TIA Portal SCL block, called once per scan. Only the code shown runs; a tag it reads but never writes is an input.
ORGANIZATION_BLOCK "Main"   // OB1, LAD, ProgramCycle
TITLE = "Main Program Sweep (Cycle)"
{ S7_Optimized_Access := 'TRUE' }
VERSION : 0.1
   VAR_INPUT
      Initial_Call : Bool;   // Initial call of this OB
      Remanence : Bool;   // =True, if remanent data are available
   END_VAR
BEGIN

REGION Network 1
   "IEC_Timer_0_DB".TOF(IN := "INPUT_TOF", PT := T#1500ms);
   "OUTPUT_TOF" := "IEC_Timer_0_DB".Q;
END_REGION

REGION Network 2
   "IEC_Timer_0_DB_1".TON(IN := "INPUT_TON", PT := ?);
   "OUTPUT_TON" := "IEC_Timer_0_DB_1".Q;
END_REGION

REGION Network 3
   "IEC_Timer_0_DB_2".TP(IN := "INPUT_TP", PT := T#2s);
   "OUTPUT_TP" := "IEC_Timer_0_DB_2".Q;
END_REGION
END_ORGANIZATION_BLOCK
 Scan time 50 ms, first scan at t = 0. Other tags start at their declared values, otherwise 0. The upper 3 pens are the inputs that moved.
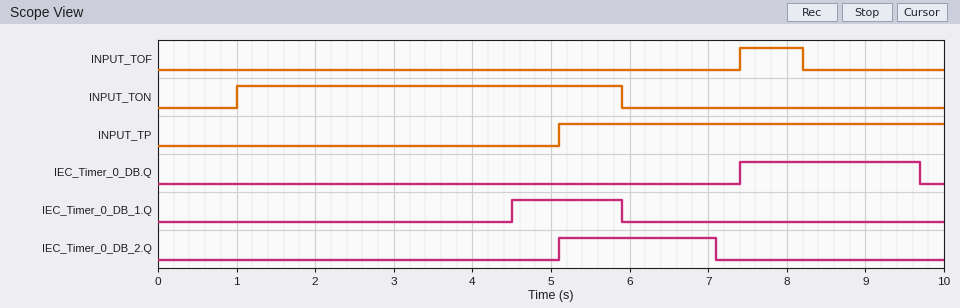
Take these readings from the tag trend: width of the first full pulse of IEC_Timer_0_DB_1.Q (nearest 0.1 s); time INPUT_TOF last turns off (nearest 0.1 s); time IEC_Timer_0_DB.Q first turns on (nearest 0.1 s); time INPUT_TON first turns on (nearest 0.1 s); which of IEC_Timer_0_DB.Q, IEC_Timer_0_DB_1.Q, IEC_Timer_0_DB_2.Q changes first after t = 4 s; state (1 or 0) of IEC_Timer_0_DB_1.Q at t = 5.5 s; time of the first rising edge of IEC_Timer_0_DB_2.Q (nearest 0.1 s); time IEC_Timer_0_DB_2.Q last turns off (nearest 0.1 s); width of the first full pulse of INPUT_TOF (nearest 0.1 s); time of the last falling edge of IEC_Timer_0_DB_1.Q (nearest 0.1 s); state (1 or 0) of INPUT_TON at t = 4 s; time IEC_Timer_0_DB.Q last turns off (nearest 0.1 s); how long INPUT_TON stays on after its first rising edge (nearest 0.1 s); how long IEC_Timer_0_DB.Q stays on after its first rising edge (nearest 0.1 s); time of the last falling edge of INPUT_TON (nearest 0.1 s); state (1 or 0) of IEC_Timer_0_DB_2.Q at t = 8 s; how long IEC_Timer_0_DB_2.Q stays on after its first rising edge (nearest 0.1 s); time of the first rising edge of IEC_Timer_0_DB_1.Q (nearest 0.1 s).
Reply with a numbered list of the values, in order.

1. 1.4 s
2. 8.2 s
3. 7.4 s
4. 1.0 s
5. IEC_Timer_0_DB_1.Q
6. 1
7. 5.1 s
8. 7.1 s
9. 0.8 s
10. 5.9 s
11. 1
12. 9.7 s
13. 4.9 s
14. 2.3 s
15. 5.9 s
16. 0
17. 2.0 s
18. 4.5 s
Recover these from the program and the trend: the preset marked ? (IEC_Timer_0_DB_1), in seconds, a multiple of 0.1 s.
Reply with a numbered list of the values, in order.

1. 3.5 s
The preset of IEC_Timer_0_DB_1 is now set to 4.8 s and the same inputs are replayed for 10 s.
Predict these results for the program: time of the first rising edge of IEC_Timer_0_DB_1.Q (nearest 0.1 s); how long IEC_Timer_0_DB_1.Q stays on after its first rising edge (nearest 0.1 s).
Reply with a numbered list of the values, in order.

1. 5.8 s
2. 0.1 s
